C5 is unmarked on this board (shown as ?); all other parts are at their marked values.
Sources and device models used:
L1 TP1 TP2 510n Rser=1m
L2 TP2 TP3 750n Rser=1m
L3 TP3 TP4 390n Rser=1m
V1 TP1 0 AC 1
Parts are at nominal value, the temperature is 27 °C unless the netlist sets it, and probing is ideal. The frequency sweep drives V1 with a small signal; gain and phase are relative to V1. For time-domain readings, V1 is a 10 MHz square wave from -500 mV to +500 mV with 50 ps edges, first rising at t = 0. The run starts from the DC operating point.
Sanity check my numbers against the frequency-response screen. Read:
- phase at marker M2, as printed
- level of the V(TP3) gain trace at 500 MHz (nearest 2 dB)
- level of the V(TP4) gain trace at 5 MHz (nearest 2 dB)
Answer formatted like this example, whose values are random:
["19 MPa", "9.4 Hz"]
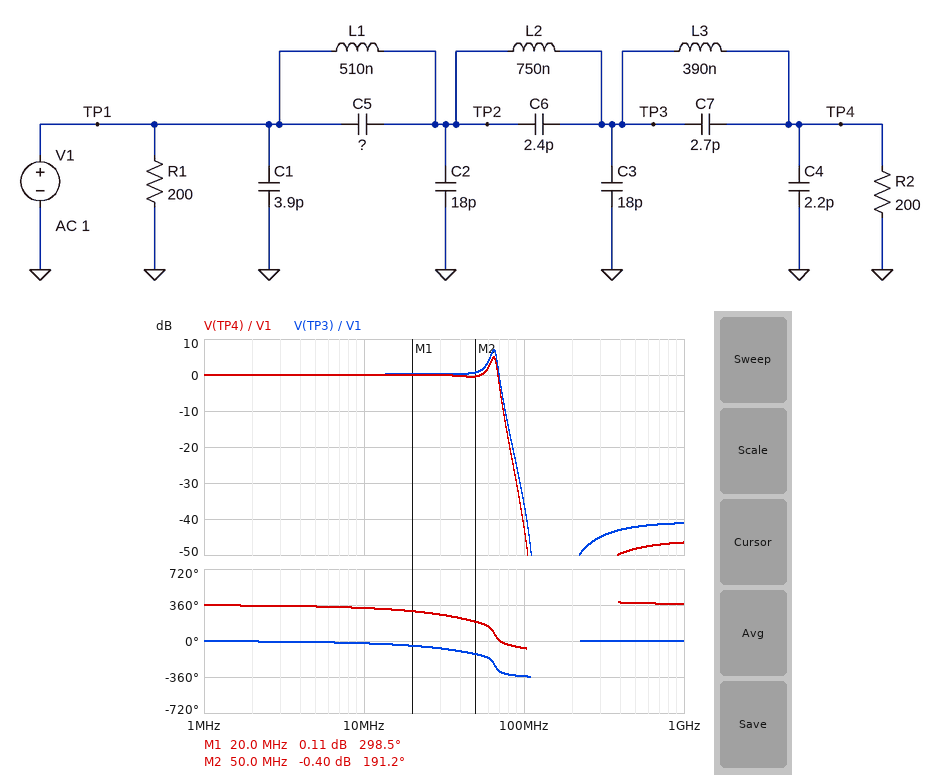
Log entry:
["191.2 deg", "-42 dB", "0 dB"]
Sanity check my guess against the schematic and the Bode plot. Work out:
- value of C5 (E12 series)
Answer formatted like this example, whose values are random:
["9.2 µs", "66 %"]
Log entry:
["1.8 pF"]
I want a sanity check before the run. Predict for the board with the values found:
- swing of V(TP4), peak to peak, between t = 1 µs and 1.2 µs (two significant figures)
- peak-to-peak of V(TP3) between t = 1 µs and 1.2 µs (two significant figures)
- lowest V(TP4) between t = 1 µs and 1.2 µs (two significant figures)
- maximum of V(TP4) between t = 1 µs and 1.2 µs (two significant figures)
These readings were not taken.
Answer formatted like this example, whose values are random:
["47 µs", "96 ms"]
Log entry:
["1.4 V", "1.5 V", "-700 mV", "700 mV"]
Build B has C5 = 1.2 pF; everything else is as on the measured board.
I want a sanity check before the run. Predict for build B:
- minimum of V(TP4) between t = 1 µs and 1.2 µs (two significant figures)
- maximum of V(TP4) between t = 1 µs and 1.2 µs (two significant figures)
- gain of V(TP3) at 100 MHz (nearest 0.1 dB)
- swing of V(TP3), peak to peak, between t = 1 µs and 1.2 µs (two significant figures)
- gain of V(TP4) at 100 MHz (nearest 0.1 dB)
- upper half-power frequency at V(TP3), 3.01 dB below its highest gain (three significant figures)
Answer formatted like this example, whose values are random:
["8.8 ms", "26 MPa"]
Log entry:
["-710 mV", "710 mV", "-33.8 dB", "1.5 V", "-40.4 dB", "68.4 MHz"]
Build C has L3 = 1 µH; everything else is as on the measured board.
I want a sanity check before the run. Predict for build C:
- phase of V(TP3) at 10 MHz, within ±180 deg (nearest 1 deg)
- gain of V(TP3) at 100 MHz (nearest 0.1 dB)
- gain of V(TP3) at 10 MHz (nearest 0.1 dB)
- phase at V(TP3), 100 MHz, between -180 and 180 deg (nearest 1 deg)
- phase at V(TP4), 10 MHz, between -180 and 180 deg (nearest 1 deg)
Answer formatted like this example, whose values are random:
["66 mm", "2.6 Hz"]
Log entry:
["-20 deg", "-37.7 dB", "-0.4 dB", "0 deg", "-38 deg"]
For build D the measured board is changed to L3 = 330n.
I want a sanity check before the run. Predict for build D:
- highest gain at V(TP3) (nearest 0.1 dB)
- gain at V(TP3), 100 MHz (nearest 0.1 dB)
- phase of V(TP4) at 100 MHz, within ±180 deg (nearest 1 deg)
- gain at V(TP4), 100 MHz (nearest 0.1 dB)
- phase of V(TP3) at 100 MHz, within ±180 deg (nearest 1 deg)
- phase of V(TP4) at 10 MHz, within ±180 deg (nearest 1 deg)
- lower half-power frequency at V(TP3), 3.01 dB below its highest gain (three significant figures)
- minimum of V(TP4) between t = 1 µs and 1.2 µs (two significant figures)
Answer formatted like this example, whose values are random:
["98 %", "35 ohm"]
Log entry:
["6.7 dB", "-35.5 dB", "-59 deg", "-40.0 dB", "12 deg", "-29 deg", "59.9 MHz", "-690 mV"]
